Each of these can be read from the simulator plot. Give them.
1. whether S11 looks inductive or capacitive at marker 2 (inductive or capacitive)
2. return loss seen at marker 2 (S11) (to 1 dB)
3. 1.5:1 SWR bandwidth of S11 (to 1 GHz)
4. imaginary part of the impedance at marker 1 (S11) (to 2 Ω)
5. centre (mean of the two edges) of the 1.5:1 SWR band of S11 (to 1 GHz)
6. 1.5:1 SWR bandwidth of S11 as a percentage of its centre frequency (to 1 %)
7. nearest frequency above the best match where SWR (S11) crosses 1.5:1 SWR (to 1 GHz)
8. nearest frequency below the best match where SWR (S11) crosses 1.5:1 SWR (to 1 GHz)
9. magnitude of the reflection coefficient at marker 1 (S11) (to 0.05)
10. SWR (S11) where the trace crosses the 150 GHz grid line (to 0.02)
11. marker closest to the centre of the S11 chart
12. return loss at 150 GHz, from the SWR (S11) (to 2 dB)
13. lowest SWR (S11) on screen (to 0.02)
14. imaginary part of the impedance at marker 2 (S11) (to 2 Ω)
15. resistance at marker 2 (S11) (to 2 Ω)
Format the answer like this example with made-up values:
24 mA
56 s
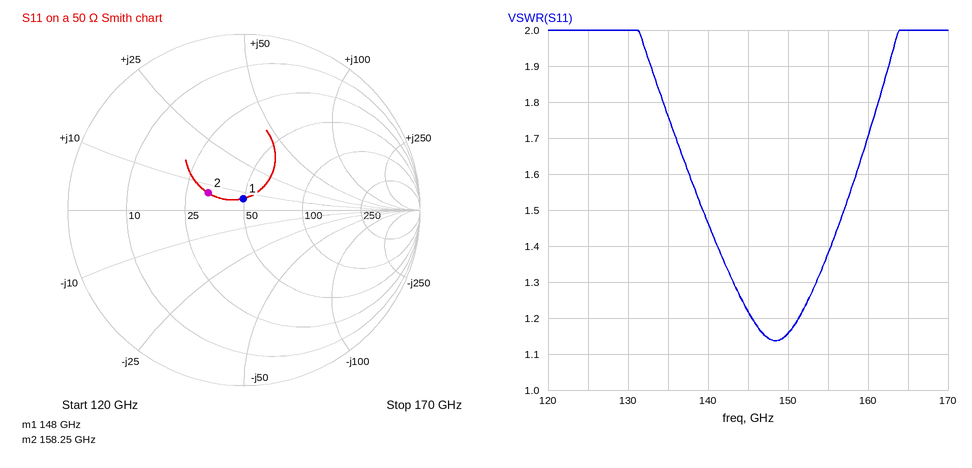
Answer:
inductive
13 dB
18 GHz
+6 Ω
148 GHz
12 %
157 GHz
139 GHz
0.05
1.16
marker 1
22 dB
1.14
+6 Ω
32 Ω
